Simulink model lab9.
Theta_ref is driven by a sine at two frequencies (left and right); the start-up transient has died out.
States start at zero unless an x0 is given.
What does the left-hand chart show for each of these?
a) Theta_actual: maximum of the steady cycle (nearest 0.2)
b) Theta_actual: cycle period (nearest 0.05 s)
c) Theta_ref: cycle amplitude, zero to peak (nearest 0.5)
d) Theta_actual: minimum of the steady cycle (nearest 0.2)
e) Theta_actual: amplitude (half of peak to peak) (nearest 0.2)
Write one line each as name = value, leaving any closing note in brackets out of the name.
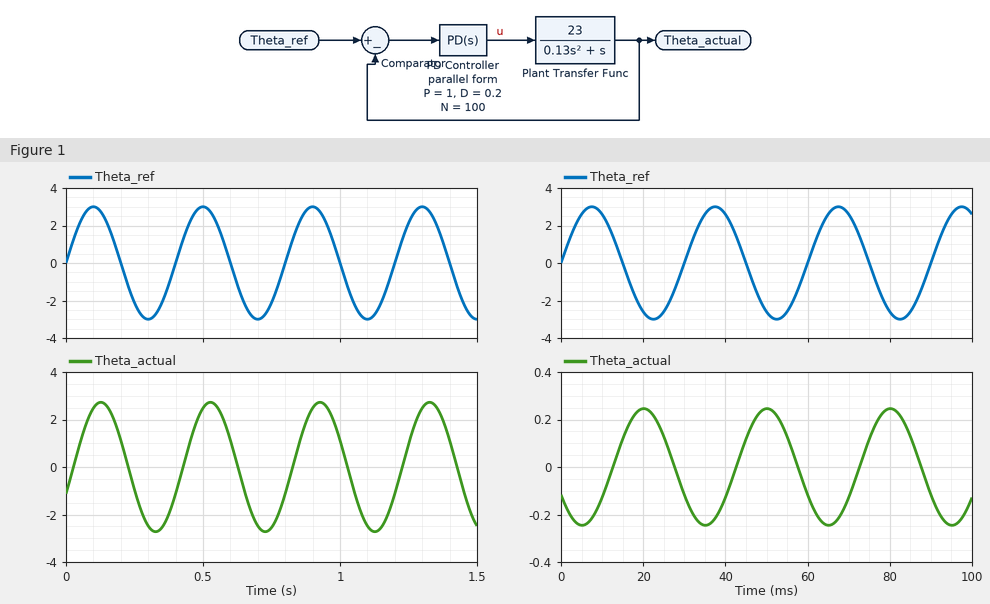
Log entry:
Theta_actual: maximum of the steady cycle = 2.8
Theta_actual: cycle period = 0.40 s
Theta_ref: cycle amplitude, zero to peak = 3.0
Theta_actual: minimum of the steady cycle = -2.8
Theta_actual: amplitude (half of peak to peak) = 2.8
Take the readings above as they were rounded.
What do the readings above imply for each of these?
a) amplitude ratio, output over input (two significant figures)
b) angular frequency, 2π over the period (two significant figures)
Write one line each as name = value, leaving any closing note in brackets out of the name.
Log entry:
amplitude ratio, output over input = 0.93
angular frequency, 2π over the period = 16 rad/s
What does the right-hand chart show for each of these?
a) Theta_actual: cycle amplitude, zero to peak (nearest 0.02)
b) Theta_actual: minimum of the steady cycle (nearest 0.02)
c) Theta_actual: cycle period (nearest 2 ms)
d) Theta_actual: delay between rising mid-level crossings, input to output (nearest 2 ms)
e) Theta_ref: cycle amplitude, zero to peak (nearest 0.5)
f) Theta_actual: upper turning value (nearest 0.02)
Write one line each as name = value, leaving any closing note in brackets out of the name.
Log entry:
Theta_actual: cycle amplitude, zero to peak = 0.24
Theta_actual: minimum of the steady cycle = -0.24
Theta_actual: cycle period = 30 ms
Theta_actual: delay between rising mid-level crossings, input to output = 12 ms
Theta_ref: cycle amplitude, zero to peak = 3.0
Theta_actual: upper turning value = 0.24
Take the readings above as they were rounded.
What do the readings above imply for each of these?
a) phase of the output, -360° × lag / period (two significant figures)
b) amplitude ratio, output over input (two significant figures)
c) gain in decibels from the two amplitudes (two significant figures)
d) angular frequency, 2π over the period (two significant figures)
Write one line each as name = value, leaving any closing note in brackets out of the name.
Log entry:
phase of the output, -360° × lag / period = -140°
amplitude ratio, output over input = 0.080
gain in decibels from the two amplitudes = -22 dB
angular frequency, 2π over the period = 0.21 rad/ms
